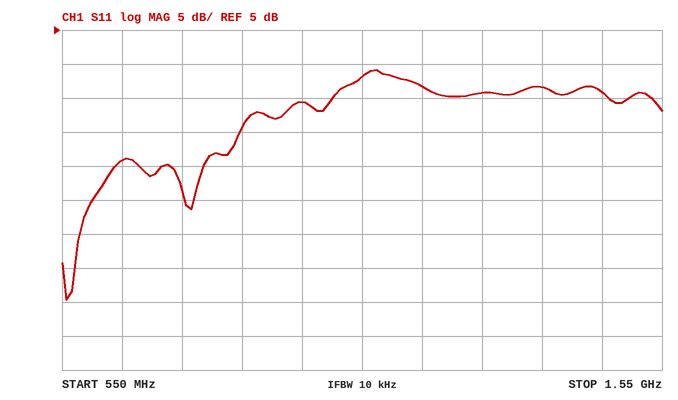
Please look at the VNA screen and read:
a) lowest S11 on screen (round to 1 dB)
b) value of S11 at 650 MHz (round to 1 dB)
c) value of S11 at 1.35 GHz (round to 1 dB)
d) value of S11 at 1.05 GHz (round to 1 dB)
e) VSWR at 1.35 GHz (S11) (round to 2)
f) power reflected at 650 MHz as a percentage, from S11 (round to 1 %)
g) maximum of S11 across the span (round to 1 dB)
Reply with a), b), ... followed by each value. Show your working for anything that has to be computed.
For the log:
a) -35 dB
b) -14 dB
c) -3 dB
d) -2 dB
e) |Γ| = 10^(-3/20) = 0.7079; VSWR = (1 + 0.7079)/(1 − 0.7079) ≈ 6
f) 10^(-14/10) ≈ 4 %
g) -1 dB
